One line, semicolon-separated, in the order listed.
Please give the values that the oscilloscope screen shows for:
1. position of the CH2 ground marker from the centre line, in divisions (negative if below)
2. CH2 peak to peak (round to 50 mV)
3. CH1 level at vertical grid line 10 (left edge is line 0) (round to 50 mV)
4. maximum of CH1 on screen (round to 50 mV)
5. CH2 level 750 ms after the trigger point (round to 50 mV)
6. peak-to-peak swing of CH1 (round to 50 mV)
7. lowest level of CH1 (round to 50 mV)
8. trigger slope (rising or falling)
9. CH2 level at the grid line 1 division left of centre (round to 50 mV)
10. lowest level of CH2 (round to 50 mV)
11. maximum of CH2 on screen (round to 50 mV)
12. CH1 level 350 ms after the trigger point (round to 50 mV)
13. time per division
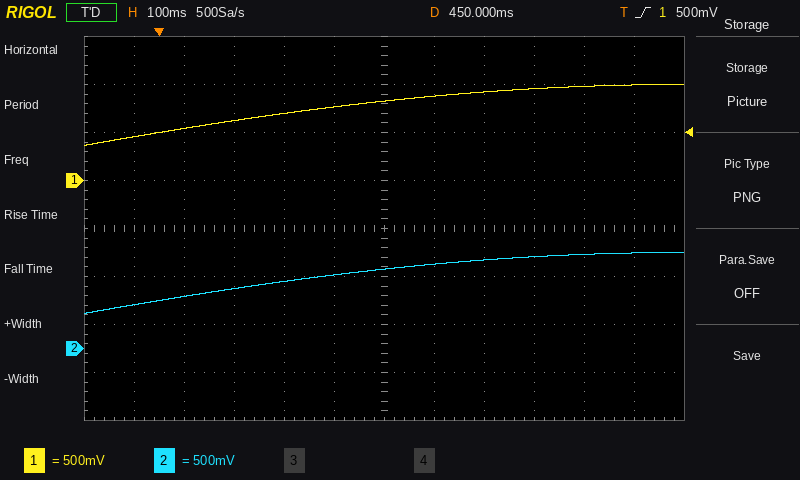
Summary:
-2.5 div; 650 mV; 1.00 V; 1.00 V; 950 mV; 650 mV; 350 mV; rising; 750 mV; 350 mV; 1.00 V; 750 mV; 100 ms
